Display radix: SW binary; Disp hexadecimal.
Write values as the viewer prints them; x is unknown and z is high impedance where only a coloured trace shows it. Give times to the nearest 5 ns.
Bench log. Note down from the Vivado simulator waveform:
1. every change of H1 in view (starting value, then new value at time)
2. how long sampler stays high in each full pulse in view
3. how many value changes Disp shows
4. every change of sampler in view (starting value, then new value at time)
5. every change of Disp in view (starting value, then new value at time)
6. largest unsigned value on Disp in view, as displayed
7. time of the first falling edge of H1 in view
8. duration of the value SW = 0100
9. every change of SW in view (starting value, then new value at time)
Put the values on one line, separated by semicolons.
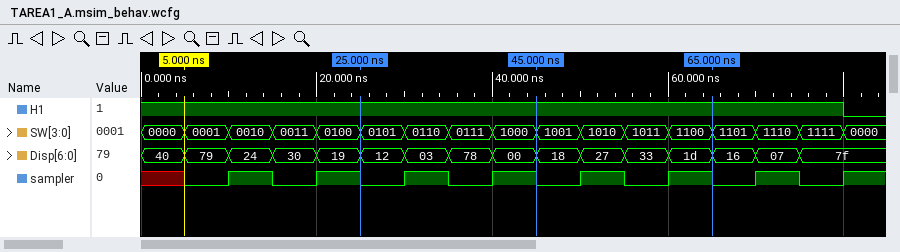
1, 0 at 80 ns; 5 ns, 5 ns, 5 ns, 5 ns, 5 ns, 5 ns, 5 ns; 15; x, 0 at 5 ns, 1 at 10 ns, 0 at 15 ns, 1 at 20 ns, 0 at 25 ns, 1 at 30 ns, 0 at 35 ns, 1 at 40 ns, 0 at 45 ns, 1 at 50 ns, 0 at 55 ns, 1 at 60 ns, 0 at 65 ns, 1 at 70 ns, 0 at 75 ns, 1 at 80 ns; 40, 79 at 5 ns, 24 at 10 ns, 30 at 15 ns, 19 at 20 ns, 12 at 25 ns, 03 at 30 ns, 78 at 35 ns, 00 at 40 ns, 18 at 45 ns, 27 at 50 ns, 33 at 55 ns, 1d at 60 ns, 16 at 65 ns, 07 at 70 ns, 7f at 75 ns; 7f; 80 ns; 5 ns; 0000, 0001 at 5 ns, 0010 at 10 ns, 0011 at 15 ns, 0100 at 20 ns, 0101 at 25 ns, 0110 at 30 ns, 0111 at 35 ns, 1000 at 40 ns, 1001 at 45 ns, 1010 at 50 ns, 1011 at 55 ns, 1100 at 60 ns, 1101 at 65 ns, 1110 at 70 ns, 1111 at 75 ns, 0000 at 80 ns
